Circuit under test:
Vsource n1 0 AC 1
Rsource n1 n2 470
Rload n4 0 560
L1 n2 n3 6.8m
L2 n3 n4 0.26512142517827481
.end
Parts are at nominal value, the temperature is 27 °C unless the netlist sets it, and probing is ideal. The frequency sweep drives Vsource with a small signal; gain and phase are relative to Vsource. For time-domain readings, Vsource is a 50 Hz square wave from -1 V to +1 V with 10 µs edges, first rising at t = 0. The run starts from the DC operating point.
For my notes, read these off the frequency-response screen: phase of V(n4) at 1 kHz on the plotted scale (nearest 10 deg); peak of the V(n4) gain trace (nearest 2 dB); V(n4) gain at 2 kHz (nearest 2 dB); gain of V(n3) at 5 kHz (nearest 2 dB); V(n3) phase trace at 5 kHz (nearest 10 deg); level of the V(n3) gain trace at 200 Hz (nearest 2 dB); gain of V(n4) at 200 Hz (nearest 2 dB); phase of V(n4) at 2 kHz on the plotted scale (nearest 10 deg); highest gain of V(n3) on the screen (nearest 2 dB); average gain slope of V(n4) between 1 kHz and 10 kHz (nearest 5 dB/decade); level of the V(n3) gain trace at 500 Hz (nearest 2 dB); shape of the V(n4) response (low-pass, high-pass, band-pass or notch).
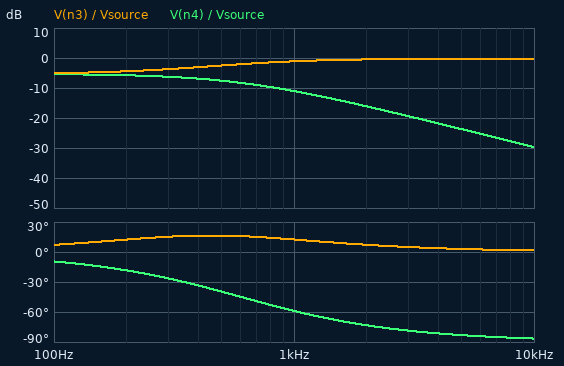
-60 deg
-6 dB
-16 dB
0 dB
0 deg
-4 dB
-6 dB
-70 deg
0 dB
-20 dB/decade
-2 dB
low-pass
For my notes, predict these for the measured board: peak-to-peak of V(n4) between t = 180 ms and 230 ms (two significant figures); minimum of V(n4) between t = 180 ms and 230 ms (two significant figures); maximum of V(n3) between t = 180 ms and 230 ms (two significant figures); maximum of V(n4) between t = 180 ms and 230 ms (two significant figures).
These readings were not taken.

1.1 V
-540 mV
1.4 V
540 mV
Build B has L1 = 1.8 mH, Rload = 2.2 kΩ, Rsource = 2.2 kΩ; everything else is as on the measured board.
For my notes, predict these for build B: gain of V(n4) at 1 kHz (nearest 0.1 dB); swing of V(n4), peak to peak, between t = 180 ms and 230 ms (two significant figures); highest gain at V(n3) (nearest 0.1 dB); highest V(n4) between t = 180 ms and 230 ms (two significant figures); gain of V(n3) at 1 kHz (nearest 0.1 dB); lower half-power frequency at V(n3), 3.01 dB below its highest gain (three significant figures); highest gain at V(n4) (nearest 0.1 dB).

-6.6 dB
1.0 V
-0.1 dB
500 mV
-4.6 dB
1.84 kHz
-6.0 dB
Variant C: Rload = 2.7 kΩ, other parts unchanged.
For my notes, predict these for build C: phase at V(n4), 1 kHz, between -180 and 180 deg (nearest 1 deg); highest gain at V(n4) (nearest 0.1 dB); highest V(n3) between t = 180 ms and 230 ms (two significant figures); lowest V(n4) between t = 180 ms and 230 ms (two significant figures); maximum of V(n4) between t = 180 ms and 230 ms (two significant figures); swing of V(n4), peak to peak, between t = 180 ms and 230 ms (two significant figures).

-28 deg
-1.4 dB
1.1 V
-850 mV
850 mV
1.7 V
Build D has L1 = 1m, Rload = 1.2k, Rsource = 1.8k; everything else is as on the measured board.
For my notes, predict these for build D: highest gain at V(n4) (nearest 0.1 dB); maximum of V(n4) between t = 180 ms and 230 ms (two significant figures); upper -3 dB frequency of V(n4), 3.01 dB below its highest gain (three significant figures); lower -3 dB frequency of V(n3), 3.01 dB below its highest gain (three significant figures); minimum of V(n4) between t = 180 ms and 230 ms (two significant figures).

-8.0 dB
400 mV
1.79 kHz
1.48 kHz
-400 mV
